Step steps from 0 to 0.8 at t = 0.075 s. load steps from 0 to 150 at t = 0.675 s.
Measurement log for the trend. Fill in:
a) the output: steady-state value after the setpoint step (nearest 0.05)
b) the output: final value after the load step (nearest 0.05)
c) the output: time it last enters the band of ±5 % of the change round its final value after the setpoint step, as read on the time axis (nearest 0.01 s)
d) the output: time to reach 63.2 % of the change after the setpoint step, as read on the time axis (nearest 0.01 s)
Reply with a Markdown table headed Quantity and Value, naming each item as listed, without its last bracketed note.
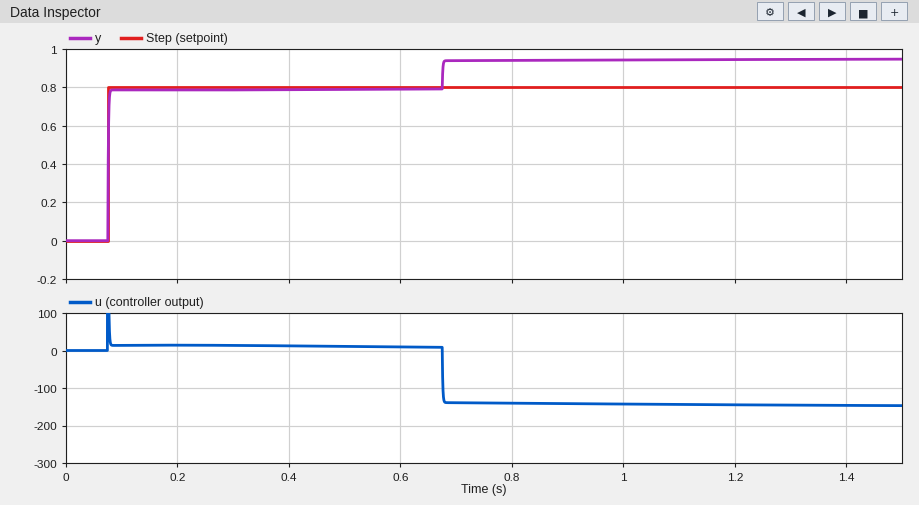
| Quantity | Value |
|---|---|
| the output: steady-state value after the setpoint step | 0.80 |
| the output: final value after the load step | 0.95 |
| the output: time it last enters the band of ±5 % of the change round its final value after the setpoint step, as read on the time axis | 0.08 s |
| the output: time to reach 63.2 % of the change after the setpoint step, as read on the time axis | 0.08 s |
